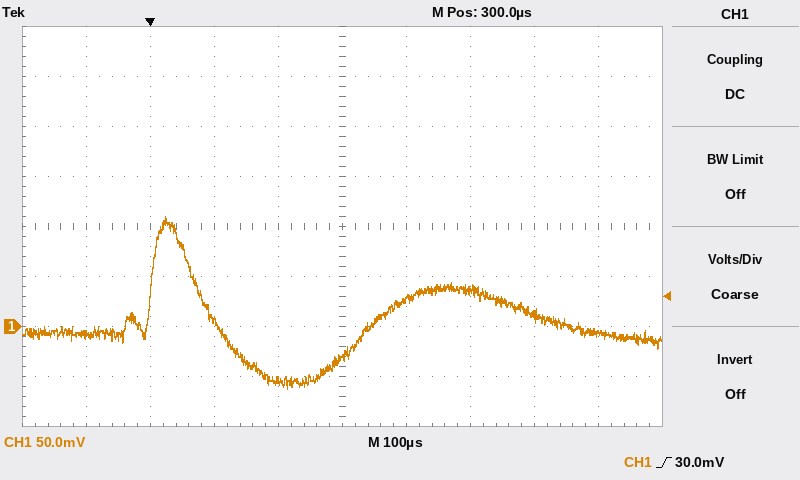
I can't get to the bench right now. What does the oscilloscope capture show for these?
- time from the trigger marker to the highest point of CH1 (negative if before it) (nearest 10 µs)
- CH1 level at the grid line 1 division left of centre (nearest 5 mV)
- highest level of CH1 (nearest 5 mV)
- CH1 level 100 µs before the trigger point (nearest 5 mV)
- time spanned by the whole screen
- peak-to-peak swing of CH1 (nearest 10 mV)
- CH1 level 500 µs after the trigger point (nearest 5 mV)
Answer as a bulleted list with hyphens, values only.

- +20 µs
- -55 mV
- 110 mV
- -10 mV
- 1 ms
- 170 mV
- 35 mV
